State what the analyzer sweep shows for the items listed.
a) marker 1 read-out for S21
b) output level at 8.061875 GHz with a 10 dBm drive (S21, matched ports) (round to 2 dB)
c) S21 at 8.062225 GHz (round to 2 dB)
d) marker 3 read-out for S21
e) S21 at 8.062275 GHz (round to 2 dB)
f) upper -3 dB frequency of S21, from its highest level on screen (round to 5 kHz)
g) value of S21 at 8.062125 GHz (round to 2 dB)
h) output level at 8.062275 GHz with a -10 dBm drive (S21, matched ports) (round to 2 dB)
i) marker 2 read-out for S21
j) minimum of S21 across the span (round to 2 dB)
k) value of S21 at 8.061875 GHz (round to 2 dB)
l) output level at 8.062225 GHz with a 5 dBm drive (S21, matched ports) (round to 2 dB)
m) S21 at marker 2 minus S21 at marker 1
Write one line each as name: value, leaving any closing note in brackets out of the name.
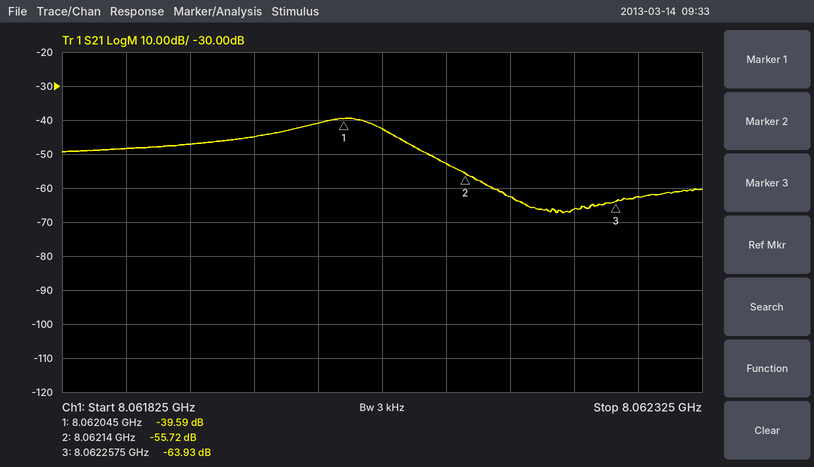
marker 1 read-out for S21: -39.59 dB
output level at 8.061875 GHz with a 10 dBm drive (S21, matched ports): -38 dBm
S21 at 8.062225 GHz: -66 dB
marker 3 read-out for S21: -63.93 dB
S21 at 8.062275 GHz: -62 dB
upper -3 dB frequency of S21, from its highest level on screen: 8.062075 GHz
value of S21 at 8.062125 GHz: -52 dB
output level at 8.062275 GHz with a -10 dBm drive (S21, matched ports): -72 dBm
marker 2 read-out for S21: -55.72 dB
minimum of S21 across the span: -68 dB
value of S21 at 8.061875 GHz: -48 dB
output level at 8.062225 GHz with a 5 dBm drive (S21, matched ports): -62 dBm
S21 at marker 2 minus S21 at marker 1: -16.13 dB
